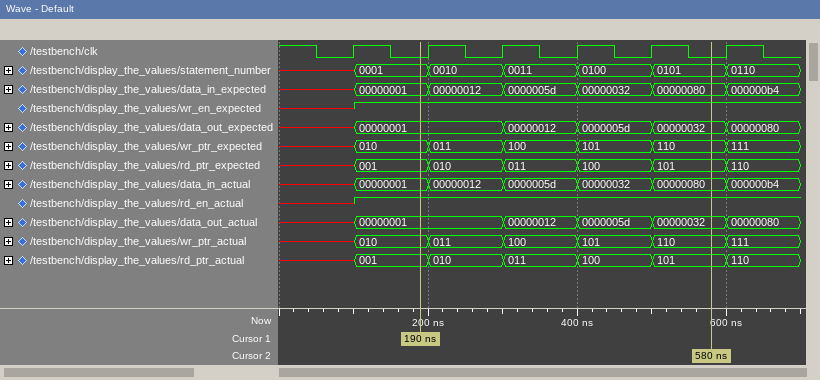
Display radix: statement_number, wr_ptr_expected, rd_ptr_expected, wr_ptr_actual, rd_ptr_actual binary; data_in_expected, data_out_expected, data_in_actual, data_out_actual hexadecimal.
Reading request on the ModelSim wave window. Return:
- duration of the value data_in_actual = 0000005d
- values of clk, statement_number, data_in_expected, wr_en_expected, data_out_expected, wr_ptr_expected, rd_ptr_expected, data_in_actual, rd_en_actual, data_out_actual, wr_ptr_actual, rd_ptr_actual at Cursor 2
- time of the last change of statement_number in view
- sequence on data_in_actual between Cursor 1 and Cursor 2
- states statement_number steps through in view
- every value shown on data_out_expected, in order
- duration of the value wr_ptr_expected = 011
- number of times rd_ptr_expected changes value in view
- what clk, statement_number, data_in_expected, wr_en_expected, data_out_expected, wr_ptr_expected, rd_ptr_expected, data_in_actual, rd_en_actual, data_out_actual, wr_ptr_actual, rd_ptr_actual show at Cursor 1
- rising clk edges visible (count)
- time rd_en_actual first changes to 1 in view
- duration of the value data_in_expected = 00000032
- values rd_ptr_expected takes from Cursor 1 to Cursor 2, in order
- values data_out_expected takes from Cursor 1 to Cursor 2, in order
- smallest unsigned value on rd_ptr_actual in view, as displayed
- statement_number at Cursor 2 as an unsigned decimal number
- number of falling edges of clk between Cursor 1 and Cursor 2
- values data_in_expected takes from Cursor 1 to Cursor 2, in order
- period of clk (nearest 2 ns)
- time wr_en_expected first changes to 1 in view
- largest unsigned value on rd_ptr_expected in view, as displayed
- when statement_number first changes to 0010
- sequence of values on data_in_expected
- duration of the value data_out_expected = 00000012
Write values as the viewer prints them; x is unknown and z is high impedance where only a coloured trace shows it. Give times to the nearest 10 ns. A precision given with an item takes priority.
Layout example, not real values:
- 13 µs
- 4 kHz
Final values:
- 100 ns
- clk=0, statement_number=0101, data_in_expected=00000080, wr_en_expected=1, data_out_expected=00000032, wr_ptr_expected=110, rd_ptr_expected=101, data_in_actual=00000080, rd_en_actual=1, data_out_actual=00000032, wr_ptr_actual=110, rd_ptr_actual=101
- 600 ns
- 00000001, 00000012, 0000005d, 00000032, 00000080
- x, 0001, 0010, 0011, 0100, 0101, 0110
- x, 00000001, 00000012, 0000005d, 00000032, 00000080
- 100 ns
- 6
- clk=0, statement_number=0001, data_in_expected=00000001, wr_en_expected=1, data_out_expected=00000001, wr_ptr_expected=010, rd_ptr_expected=001, data_in_actual=00000001, rd_en_actual=1, data_out_actual=00000001, wr_ptr_actual=010, rd_ptr_actual=001
- 6
- 100 ns
- 100 ns
- 001, 010, 011, 100, 101
- 00000001, 00000012, 0000005d, 00000032
- 001
- 5
- 4
- 00000001, 00000012, 0000005d, 00000032, 00000080
- 100 ns
- 100 ns
- 110
- 200 ns
- x, 00000001, 00000012, 0000005d, 00000032, 00000080, 000000b4
- 100 ns
